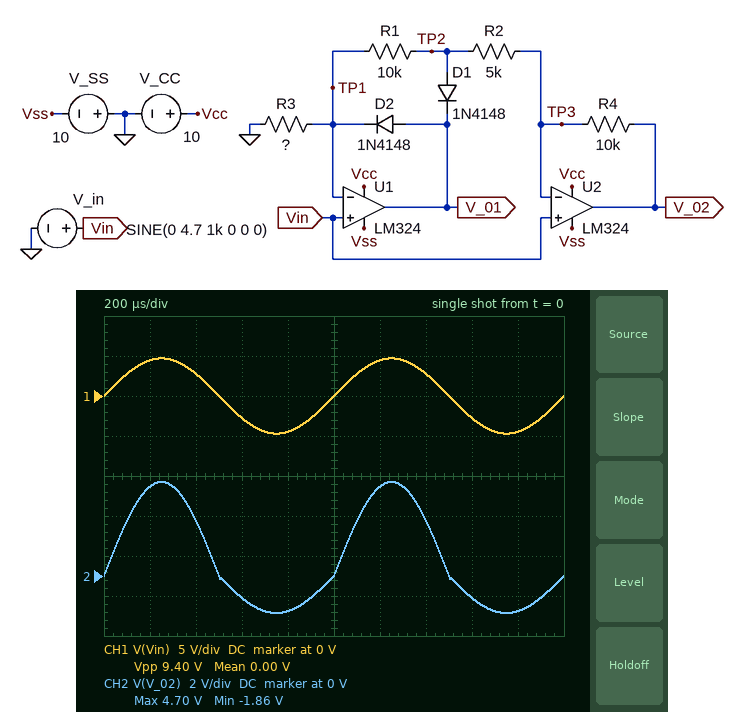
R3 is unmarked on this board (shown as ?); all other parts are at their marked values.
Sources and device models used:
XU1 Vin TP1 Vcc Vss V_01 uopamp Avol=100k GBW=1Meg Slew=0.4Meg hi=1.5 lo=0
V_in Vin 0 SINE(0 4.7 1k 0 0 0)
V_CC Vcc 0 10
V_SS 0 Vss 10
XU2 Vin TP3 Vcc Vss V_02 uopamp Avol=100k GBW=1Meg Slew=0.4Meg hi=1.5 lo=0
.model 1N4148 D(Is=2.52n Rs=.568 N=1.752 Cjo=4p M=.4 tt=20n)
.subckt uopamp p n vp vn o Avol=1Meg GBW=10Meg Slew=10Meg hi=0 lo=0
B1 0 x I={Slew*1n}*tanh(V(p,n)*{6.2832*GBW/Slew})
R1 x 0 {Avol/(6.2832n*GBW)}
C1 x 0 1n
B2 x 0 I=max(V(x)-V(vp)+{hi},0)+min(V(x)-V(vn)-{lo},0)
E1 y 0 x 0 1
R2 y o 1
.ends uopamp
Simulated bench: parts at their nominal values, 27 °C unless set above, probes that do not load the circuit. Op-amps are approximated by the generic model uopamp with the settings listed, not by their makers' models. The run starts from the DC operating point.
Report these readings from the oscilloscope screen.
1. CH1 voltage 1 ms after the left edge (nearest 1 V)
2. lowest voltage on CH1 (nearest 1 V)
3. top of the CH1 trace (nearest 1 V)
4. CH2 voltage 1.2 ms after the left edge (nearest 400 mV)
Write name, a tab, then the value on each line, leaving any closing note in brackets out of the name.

CH1 voltage 1 ms after the left edge	0 V
lowest voltage on CH1	-5 V
top of the CH1 trace	5 V
CH2 voltage 1.2 ms after the left edge	4.4 V
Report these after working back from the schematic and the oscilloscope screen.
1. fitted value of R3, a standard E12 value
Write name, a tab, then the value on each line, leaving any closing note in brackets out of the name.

fitted value of R3, a standard E12 value	33 kΩ
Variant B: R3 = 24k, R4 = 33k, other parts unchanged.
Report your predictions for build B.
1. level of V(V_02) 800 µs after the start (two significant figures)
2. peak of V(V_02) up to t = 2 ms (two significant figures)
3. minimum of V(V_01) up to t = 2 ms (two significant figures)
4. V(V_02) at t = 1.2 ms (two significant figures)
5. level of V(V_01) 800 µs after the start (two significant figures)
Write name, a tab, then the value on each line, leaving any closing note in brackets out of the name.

level of V(V_02) 800 µs after the start	7.9 V
peak of V(V_02) up to t = 2 ms	8.2 V
minimum of V(V_01) up to t = 2 ms	-7.2 V
V(V_02) at t = 1.2 ms	4.5 V
level of V(V_01) 800 µs after the start	-6.9 V
